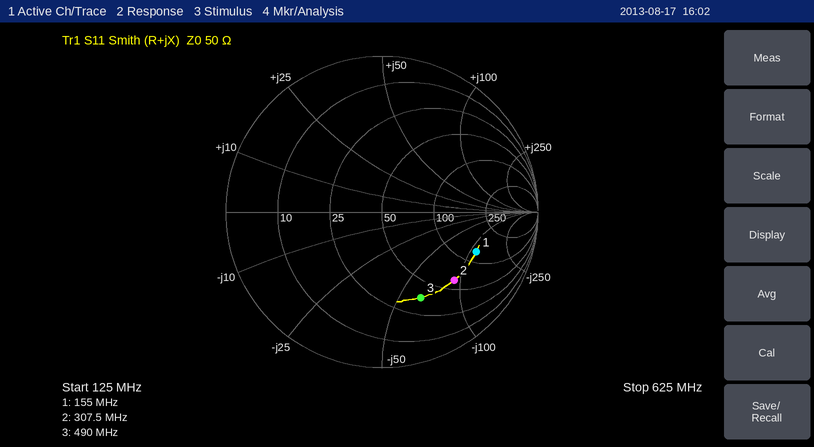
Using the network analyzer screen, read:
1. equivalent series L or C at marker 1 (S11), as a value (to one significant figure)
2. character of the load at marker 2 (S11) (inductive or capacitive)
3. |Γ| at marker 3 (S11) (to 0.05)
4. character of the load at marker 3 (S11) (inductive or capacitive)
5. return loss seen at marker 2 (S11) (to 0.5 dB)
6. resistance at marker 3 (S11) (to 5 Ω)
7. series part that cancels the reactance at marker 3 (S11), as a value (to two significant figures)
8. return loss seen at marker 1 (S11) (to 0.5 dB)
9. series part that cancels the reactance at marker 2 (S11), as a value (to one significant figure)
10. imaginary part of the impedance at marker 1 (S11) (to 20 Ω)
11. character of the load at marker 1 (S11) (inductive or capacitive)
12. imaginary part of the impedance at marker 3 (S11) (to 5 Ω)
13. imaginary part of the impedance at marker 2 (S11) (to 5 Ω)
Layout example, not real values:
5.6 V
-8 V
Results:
9 pF
capacitive
0.60
capacitive
4.0 dB
35 Ω
21 nH
3.5 dB
50 nH
-120 Ω
capacitive
-65 Ω
-90 Ω
